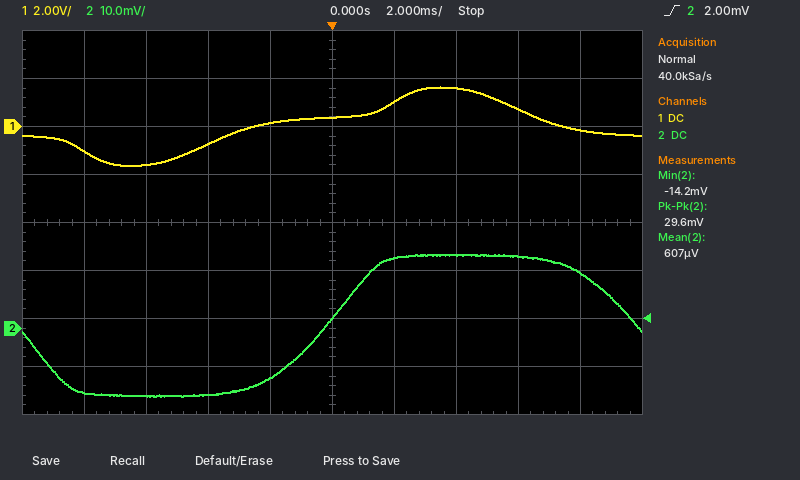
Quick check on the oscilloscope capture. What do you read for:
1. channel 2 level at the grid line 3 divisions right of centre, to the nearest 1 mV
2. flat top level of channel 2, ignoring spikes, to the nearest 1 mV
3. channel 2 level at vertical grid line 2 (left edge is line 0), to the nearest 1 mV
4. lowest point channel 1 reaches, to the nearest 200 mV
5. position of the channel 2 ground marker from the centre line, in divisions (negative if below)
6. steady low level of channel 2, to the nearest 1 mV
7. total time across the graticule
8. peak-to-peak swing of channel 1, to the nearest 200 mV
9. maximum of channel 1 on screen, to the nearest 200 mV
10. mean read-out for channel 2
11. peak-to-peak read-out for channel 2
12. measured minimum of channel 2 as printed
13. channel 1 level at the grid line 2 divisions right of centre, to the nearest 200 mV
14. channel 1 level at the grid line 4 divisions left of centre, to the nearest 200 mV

15 mV
15 mV
-14 mV
-1.6 V
-2.2 div
-14 mV
20 ms
3.2 V
1.6 V
607 µV
29.6 mV
-14.2 mV
1.6 V
-1.0 V
